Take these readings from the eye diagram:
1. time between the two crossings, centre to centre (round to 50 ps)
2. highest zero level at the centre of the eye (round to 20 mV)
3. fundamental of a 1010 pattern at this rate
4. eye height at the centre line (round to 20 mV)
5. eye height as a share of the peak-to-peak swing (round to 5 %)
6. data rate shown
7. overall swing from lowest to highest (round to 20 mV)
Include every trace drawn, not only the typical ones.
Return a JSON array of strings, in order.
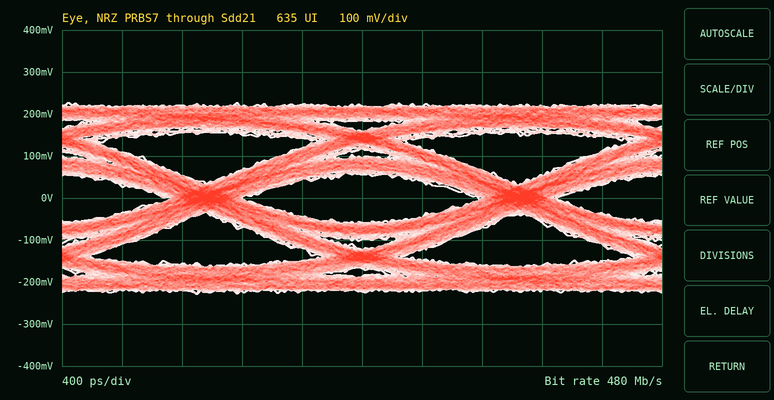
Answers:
["2.10 ns", "-60 mV", "240 MHz", "120 mV", "25 %", "480 Mb/s", "460 mV"]
